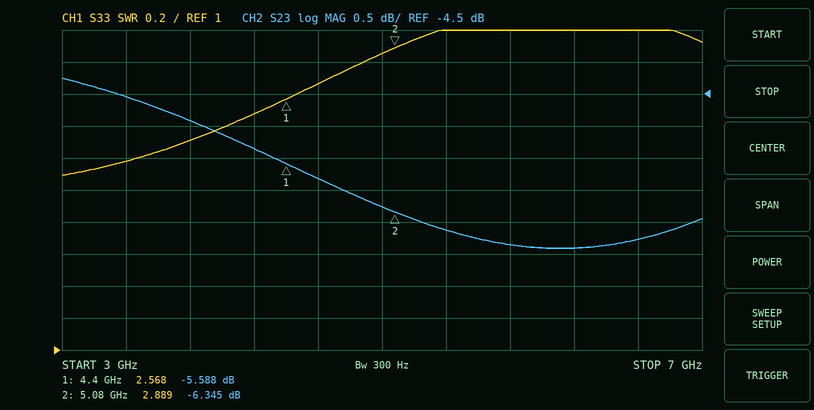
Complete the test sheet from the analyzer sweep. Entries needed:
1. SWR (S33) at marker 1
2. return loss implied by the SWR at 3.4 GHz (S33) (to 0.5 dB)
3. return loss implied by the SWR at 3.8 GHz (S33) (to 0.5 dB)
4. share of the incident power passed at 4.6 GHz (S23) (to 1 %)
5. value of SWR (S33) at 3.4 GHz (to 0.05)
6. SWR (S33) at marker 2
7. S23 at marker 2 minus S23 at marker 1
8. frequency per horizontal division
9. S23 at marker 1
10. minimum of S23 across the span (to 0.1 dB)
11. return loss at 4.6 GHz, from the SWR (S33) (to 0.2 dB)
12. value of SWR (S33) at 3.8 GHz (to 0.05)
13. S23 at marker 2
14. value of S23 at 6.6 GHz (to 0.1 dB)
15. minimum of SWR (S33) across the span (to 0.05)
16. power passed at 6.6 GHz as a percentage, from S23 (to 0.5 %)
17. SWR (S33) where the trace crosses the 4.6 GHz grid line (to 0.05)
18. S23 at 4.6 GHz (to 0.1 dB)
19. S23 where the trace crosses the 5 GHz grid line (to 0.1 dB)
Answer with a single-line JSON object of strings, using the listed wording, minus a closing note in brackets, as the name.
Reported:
{"SWR (S33) at marker 1": "2.568", "return loss implied by the SWR at 3.4 GHz (S33)": "8.5 dB", "return loss implied by the SWR at 3.8 GHz (S33)": "8.0 dB", "share of the incident power passed at 4.6 GHz (S23)": "26 %", "value of SWR (S33) at 3.4 GHz": "2.20", "SWR (S33) at marker 2": "2.889", "S23 at marker 2 minus S23 at marker 1": "-0.757 dB", "frequency per horizontal division": "400 MHz", "S23 at marker 1": "-5.588 dB", "minimum of S23 across the span": "-6.9 dB", "return loss at 4.6 GHz, from the SWR (S33)": "6.8 dB", "value of SWR (S33) at 3.8 GHz": "2.30", "S23 at marker 2": "-6.345 dB", "value of S23 at 6.6 GHz": "-6.8 dB", "minimum of SWR (S33) across the span": "2.10", "power passed at 6.6 GHz as a percentage, from S23": "21.0 %", "SWR (S33) where the trace crosses the 4.6 GHz grid line": "2.65", "S23 at 4.6 GHz": "-5.8 dB", "S23 where the trace crosses the 5 GHz grid line": "-6.3 dB"}
